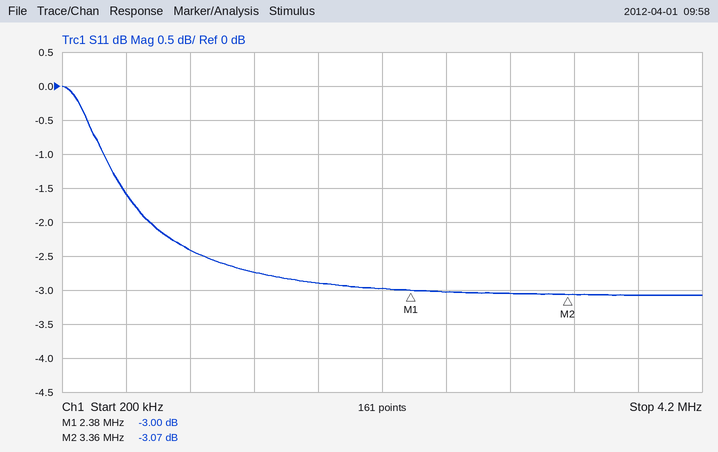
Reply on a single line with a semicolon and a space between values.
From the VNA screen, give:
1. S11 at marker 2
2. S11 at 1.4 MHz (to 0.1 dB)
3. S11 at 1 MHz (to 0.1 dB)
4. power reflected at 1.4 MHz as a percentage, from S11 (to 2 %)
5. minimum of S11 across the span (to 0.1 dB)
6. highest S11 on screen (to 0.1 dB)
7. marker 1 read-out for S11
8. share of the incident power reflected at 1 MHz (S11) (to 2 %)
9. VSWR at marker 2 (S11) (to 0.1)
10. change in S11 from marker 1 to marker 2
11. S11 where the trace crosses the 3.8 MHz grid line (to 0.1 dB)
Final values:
-3.07 dB; -2.7 dB; -2.4 dB; 54 %; -3.1 dB; 0.0 dB; -3.00 dB; 58 %; 5.7; -0.07 dB; -3.1 dB
